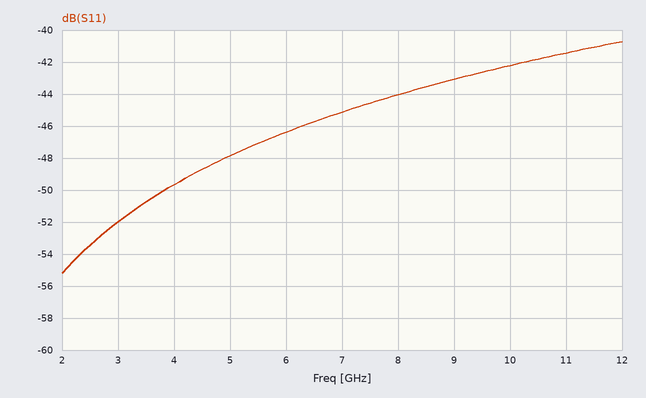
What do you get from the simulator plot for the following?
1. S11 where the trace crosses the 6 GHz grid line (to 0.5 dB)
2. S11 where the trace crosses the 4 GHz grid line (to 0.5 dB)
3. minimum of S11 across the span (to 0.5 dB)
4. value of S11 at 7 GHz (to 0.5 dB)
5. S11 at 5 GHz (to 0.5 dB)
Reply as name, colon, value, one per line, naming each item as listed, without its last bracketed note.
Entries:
S11 where the trace crosses the 6 GHz grid line: -46.5 dB
S11 where the trace crosses the 4 GHz grid line: -49.5 dB
minimum of S11 across the span: -55.0 dB
value of S11 at 7 GHz: -45.0 dB
S11 at 5 GHz: -48.0 dB
